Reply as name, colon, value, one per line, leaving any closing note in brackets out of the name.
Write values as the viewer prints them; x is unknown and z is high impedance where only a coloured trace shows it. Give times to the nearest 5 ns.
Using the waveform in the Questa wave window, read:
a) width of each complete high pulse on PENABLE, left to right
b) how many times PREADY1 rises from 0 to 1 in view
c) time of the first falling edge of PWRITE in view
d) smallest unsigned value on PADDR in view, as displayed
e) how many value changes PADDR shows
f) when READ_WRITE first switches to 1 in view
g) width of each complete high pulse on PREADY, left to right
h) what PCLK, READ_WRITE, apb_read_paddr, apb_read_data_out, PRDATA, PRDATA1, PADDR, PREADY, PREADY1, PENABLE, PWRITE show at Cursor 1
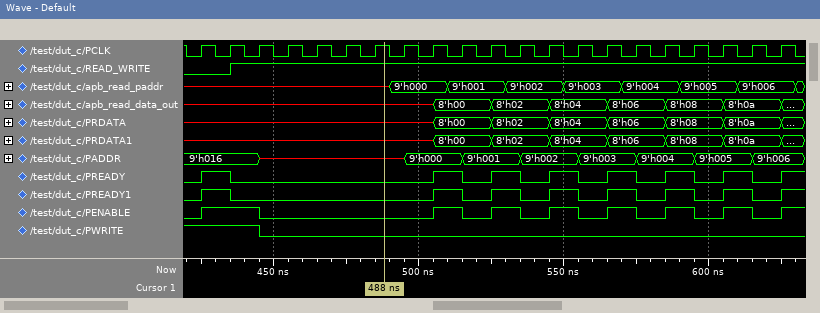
width of each complete high pulse on PENABLE, left to right: 20 ns, 10 ns, 10 ns, 10 ns, 10 ns, 10 ns, 10 ns
how many times PREADY1 rises from 0 to 1 in view: 8
time of the first falling edge of PWRITE in view: 445 ns
smallest unsigned value on PADDR in view, as displayed: 9'h000
how many value changes PADDR shows: 8
when READ_WRITE first switches to 1 in view: 435 ns
width of each complete high pulse on PREADY, left to right: 10 ns, 10 ns, 10 ns, 10 ns, 10 ns, 10 ns, 10 ns
what PCLK, READ_WRITE, apb_read_paddr, apb_read_data_out, PRDATA, PRDATA1, PADDR, PREADY, PREADY1, PENABLE, PWRITE show at Cursor 1: PCLK=1, READ_WRITE=1, apb_read_paddr=x, apb_read_data_out=x, PRDATA=x, PRDATA1=x, PADDR=x, PREADY=0, PREADY1=0, PENABLE=0, PWRITE=0
